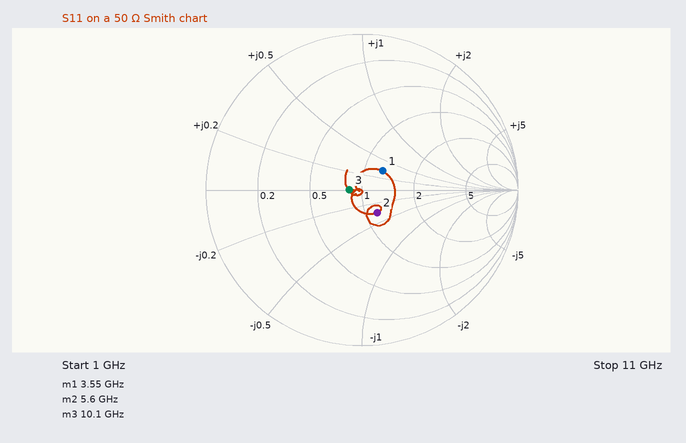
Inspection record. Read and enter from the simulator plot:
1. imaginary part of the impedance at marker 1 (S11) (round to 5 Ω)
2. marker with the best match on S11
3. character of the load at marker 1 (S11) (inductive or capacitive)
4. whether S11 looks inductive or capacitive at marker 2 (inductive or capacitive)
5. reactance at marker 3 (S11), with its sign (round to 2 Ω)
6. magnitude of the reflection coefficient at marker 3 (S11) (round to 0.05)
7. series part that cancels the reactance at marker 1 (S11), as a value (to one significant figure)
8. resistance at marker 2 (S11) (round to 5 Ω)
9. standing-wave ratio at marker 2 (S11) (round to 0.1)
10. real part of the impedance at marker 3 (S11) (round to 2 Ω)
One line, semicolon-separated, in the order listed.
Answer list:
+15 Ω; marker 3; inductive; capacitive; 0 Ω; 0.10; 3 pF; 60 Ω; 1.4; 42 Ω
